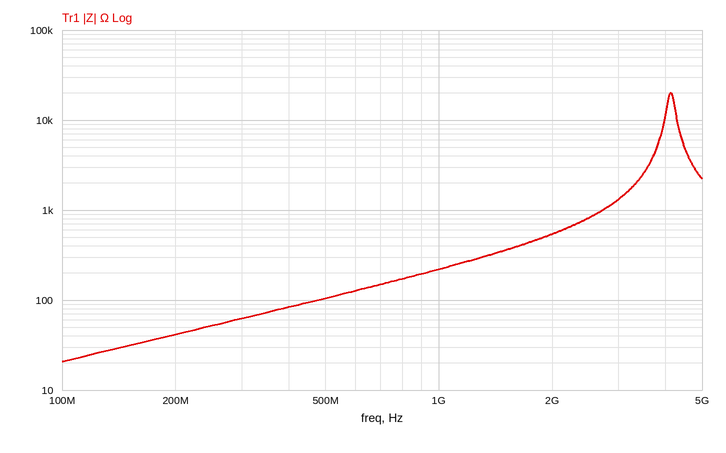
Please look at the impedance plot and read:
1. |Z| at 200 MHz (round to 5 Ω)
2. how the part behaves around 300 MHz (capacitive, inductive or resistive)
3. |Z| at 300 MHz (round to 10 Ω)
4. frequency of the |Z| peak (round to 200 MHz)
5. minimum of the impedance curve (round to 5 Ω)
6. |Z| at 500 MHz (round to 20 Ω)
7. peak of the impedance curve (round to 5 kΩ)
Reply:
40 Ω
inductive
60 Ω
4.2 GHz
20 Ω
100 Ω
20 kΩ
